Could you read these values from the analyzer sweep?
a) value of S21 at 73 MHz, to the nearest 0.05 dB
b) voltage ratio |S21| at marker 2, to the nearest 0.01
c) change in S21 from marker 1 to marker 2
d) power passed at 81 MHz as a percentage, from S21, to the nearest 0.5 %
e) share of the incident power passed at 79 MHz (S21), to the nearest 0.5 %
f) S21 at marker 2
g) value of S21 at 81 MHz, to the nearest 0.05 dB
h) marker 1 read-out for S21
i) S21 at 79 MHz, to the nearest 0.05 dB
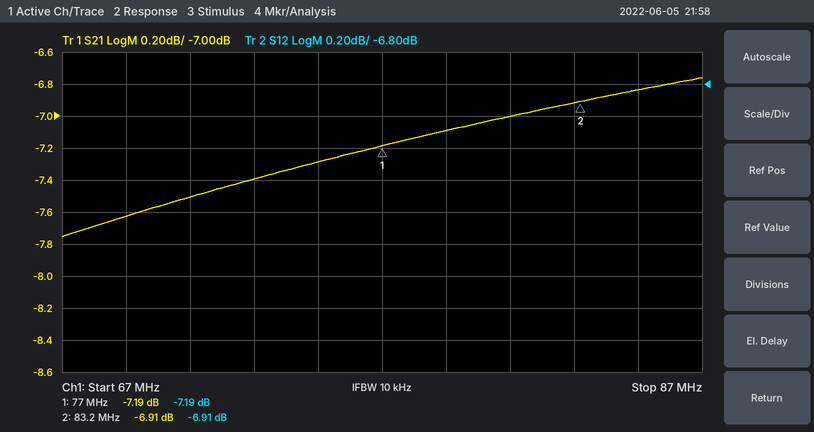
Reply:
-7.40 dB
0.45
0.28 dB
20.0 %
19.5 %
-6.91 dB
-7.00 dB
-7.19 dB
-7.10 dB
